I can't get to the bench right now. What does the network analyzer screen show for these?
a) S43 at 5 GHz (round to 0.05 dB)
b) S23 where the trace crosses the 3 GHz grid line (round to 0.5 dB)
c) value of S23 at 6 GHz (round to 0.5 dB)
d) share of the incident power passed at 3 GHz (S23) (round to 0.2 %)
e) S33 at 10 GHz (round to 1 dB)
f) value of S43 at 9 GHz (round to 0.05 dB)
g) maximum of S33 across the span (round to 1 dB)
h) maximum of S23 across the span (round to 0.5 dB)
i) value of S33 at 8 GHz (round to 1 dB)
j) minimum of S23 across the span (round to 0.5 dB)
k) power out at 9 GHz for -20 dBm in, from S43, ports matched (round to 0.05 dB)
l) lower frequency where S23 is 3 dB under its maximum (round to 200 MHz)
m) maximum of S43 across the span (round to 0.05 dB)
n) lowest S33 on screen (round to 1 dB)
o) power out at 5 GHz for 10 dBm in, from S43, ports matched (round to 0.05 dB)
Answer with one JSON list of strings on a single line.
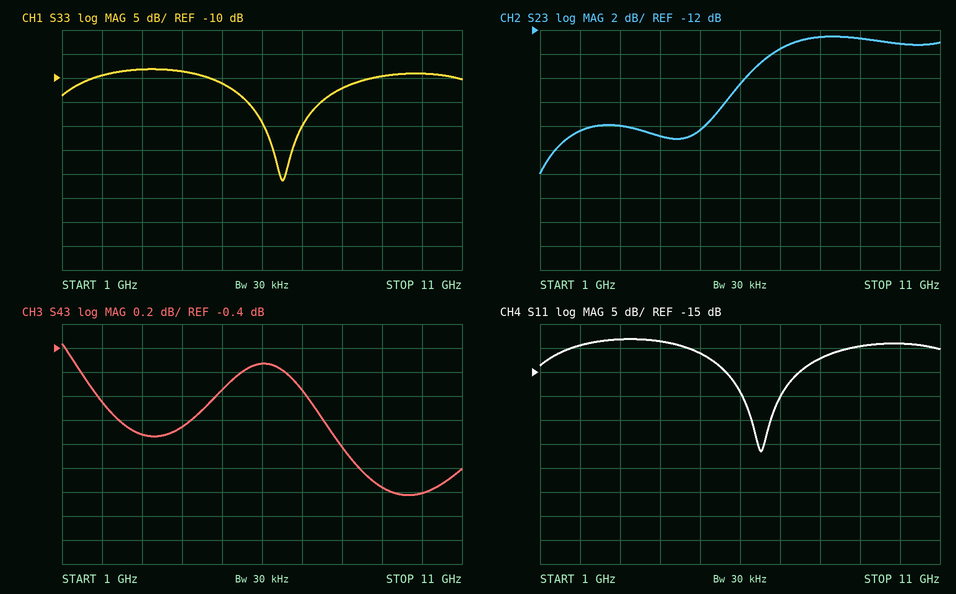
["-0.75 dB", "-20.0 dB", "-16.5 dB", "1.0 %", "-9 dB", "-1.55 dB", "-8 dB", "-12.5 dB", "-12 dB", "-24.0 dB", "-21.55 dBm", "6.2 GHz", "-0.35 dB", "-31 dB", "9.25 dBm"]
